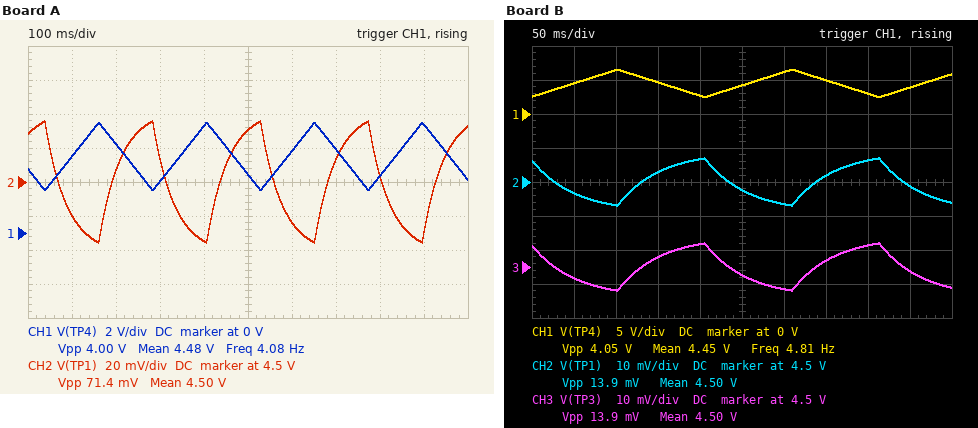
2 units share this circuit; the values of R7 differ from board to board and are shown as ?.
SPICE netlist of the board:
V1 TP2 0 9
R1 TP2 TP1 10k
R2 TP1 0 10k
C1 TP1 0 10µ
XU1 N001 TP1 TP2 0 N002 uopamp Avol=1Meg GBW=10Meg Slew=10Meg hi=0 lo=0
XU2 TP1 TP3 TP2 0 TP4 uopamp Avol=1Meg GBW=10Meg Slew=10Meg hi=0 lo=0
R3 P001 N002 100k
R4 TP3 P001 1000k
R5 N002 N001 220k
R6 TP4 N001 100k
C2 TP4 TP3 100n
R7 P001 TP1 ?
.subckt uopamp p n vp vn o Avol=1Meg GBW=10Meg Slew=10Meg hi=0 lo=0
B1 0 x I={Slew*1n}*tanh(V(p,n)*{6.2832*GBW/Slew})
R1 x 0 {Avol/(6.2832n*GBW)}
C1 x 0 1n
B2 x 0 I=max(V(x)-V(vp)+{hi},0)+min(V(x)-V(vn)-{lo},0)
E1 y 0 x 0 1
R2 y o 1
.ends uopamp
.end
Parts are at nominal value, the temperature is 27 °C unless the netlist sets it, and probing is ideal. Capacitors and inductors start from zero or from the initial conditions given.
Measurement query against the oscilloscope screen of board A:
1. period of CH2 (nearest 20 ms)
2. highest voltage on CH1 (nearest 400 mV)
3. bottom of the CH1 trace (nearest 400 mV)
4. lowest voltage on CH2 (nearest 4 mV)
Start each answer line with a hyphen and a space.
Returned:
- 240 ms
- 6.4 V
- 2.4 V
- 4.464 V
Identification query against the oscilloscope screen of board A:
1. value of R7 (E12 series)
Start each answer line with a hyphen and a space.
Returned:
- 390 kΩ
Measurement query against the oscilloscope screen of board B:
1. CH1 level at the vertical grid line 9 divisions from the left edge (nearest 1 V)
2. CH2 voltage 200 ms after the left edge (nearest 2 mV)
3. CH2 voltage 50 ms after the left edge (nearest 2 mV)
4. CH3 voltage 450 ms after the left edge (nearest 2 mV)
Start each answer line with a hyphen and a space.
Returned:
- 4 V
- 4.506 V
- 4.496 V
- 4.498 V
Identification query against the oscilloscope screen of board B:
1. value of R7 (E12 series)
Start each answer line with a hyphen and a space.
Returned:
- 2.2 MΩ
